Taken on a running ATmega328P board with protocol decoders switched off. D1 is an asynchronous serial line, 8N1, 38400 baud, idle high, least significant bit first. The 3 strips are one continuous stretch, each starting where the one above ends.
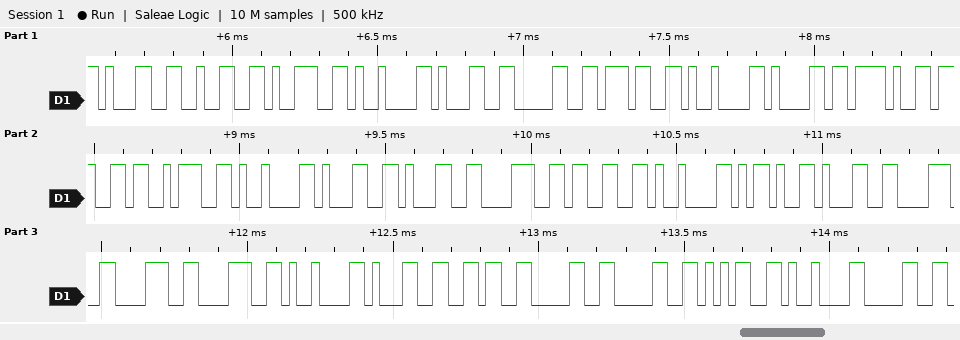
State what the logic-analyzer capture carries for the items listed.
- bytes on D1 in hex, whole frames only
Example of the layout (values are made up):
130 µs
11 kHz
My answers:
31 32 39 09 31 30 37 09 61 2F 67 3A 09 31 31 38 33 09 2D 31 38 38 38 09 31 36 30 30 35 09 30
